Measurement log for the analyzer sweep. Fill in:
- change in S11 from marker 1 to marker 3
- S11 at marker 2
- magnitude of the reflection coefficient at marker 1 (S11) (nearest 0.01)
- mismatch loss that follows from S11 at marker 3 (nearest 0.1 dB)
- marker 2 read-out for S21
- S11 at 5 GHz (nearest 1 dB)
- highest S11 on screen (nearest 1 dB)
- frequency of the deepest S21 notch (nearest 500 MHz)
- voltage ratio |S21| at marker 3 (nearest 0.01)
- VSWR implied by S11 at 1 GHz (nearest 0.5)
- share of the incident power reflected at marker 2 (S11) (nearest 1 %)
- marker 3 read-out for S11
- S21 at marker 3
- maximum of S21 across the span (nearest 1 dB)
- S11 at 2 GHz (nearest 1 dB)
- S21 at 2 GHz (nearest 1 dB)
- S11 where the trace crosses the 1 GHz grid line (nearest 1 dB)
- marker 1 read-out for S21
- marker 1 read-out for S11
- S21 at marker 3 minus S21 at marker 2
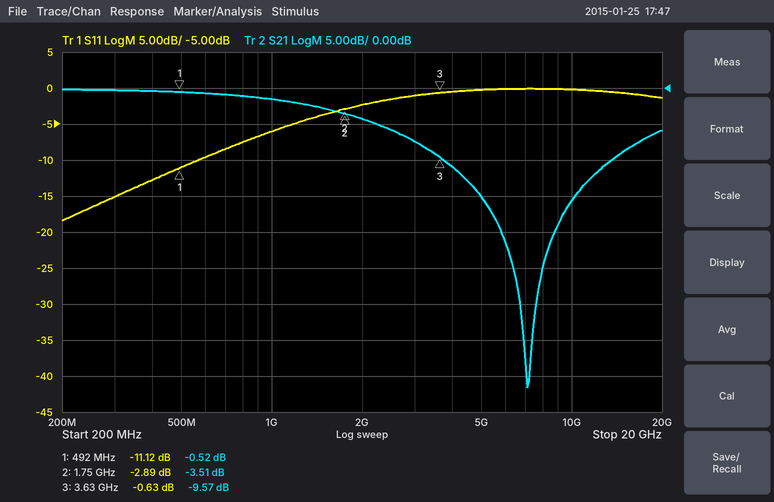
10.49 dB
-2.89 dB
0.28
8.7 dB
-3.51 dB
0 dB
0 dB
7.0 GHz
0.33
3.0
51 %
-0.63 dB
-9.57 dB
0 dB
-2 dB
-4 dB
-6 dB
-0.52 dB
-11.12 dB
-6.06 dB
